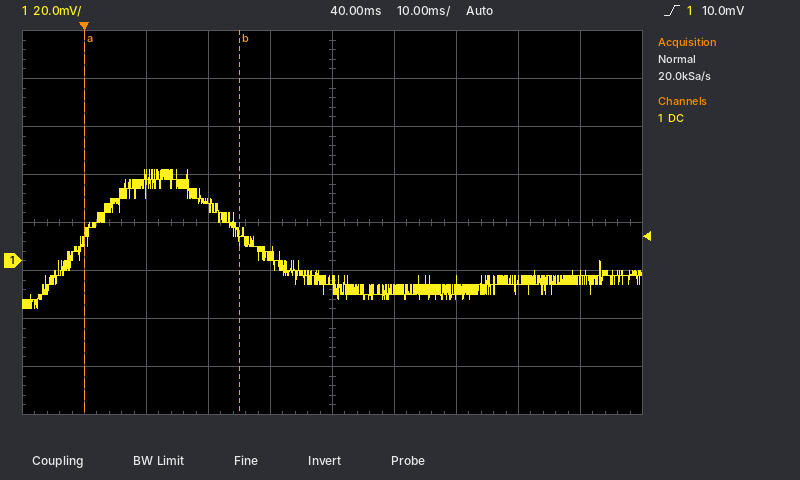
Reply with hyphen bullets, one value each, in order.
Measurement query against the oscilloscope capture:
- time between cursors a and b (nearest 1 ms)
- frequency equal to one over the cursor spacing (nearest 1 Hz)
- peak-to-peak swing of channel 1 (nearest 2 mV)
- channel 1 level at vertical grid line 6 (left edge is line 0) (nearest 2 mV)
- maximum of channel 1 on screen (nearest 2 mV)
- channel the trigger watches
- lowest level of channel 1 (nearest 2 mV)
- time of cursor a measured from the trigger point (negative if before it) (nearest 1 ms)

- 25 ms
- 40 Hz
- 58 mV
- -12 mV
- 38 mV
- channel 1
- -20 mV
- 0 ms
